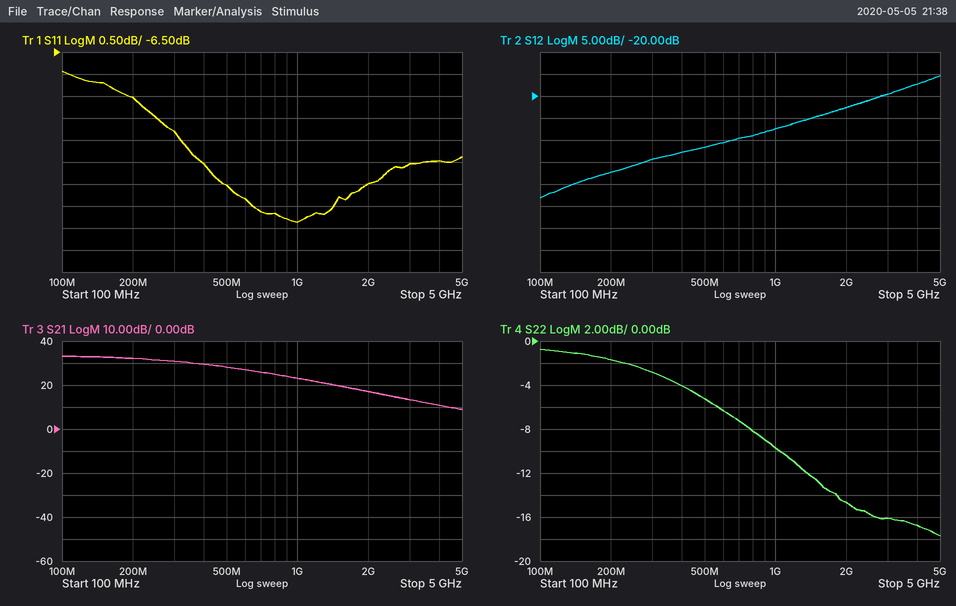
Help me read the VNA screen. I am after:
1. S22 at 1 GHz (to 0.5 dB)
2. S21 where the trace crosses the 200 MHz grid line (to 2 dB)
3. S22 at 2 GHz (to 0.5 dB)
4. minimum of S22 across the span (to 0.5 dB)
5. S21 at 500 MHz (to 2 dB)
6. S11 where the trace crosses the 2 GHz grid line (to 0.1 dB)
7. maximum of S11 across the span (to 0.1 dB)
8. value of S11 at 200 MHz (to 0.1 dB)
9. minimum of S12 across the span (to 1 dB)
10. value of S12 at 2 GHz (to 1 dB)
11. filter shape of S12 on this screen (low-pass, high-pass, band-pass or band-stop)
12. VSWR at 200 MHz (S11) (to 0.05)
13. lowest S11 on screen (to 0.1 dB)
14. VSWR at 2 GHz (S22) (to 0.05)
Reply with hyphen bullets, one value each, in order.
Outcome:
- -9.5 dB
- 32 dB
- -14.5 dB
- -17.5 dB
- 28 dB
- -9.5 dB
- -6.9 dB
- -7.5 dB
- -43 dB
- -23 dB
- high-pass
- 2.45
- -10.4 dB
- 1.45
